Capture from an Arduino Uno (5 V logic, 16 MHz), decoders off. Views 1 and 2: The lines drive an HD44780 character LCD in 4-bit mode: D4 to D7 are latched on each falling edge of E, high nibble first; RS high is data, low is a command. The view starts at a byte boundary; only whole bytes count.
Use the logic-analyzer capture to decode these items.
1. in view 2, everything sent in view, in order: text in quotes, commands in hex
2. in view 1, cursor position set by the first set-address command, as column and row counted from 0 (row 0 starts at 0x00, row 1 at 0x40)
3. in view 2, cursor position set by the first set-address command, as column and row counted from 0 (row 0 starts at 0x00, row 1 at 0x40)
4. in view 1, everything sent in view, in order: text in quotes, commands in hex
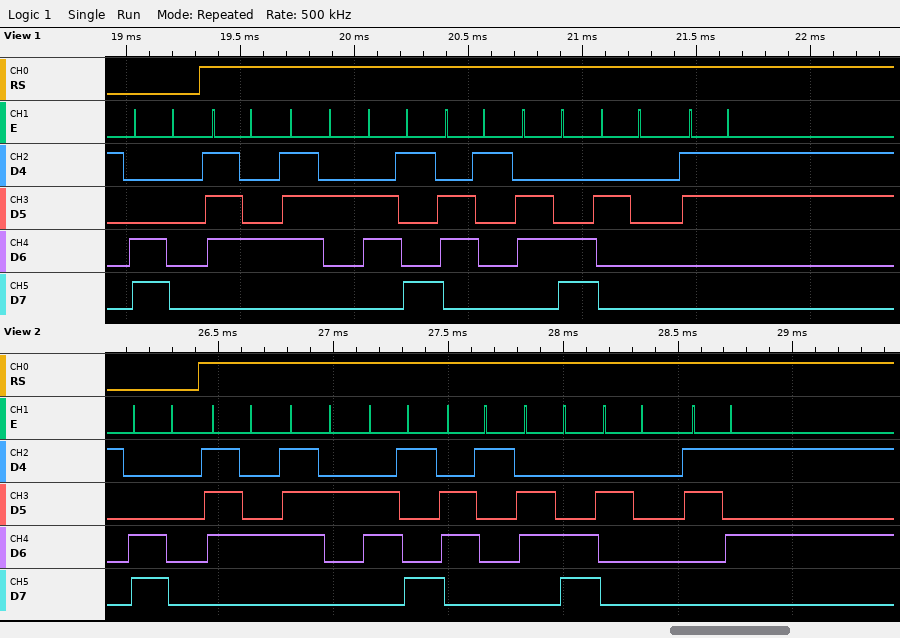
0xC0 "trial 5"
column 0, row 1
column 0, row 1
0xC0 "trial 3"
